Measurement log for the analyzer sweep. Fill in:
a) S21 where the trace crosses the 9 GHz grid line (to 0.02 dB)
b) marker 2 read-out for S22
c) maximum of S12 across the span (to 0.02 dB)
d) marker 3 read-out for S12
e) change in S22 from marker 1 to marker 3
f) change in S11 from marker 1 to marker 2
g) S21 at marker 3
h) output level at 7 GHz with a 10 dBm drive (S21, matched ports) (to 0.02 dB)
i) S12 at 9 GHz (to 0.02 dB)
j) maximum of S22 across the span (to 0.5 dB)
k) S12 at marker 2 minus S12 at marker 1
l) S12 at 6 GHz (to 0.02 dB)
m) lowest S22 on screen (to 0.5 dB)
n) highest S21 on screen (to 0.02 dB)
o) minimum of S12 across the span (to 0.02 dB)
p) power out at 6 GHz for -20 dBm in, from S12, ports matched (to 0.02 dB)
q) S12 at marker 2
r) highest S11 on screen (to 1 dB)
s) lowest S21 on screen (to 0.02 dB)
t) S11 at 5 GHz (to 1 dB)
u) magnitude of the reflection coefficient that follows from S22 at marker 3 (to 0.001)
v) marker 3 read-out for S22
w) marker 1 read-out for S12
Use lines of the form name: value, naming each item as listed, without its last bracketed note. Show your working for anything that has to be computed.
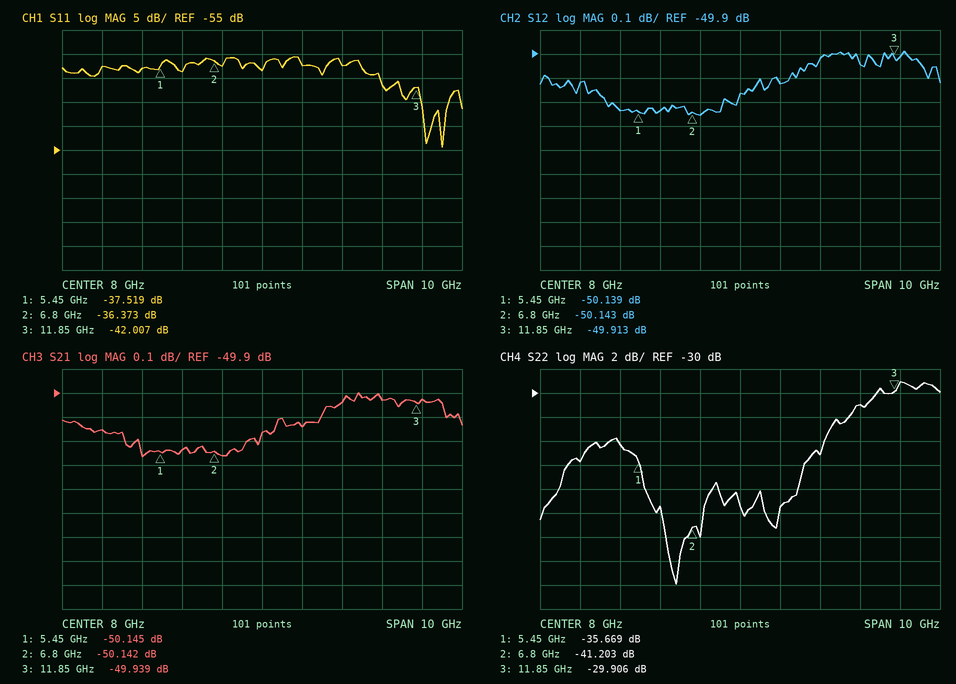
S21 where the trace crosses the 9 GHz grid line: -50.04 dB
marker 2 read-out for S22: -41.203 dB
maximum of S12 across the span: -49.88 dB
marker 3 read-out for S12: -49.913 dB
change in S22 from marker 1 to marker 3: -29.906 − (-35.669) = 5.763 dB
change in S11 from marker 1 to marker 2: -36.373 − (-37.519) = 1.146 dB
S21 at marker 3: -49.939 dB
output level at 7 GHz with a 10 dBm drive (S21, matched ports): 10 dBm + (-50.16 dB) = -40.16 dBm
S12 at 9 GHz: -50.02 dB
maximum of S22 across the span: -29.0 dB
S12 at marker 2 minus S12 at marker 1: -50.143 − (-50.139) = -0.004 dB
S12 at 6 GHz: -50.14 dB
lowest S22 on screen: -46.0 dB
highest S21 on screen: -49.90 dB
minimum of S12 across the span: -50.16 dB
power out at 6 GHz for -20 dBm in, from S12, ports matched: -20 dBm + (-50.14 dB) = -70.14 dBm
S12 at marker 2: -50.143 dB
highest S11 on screen: -36 dB
lowest S21 on screen: -50.16 dB
S11 at 5 GHz: -38 dB
magnitude of the reflection coefficient that follows from S22 at marker 3: 10^(-29.906/20) ≈ 0.032
marker 3 read-out for S22: -29.906 dB
marker 1 read-out for S12: -50.139 dB
